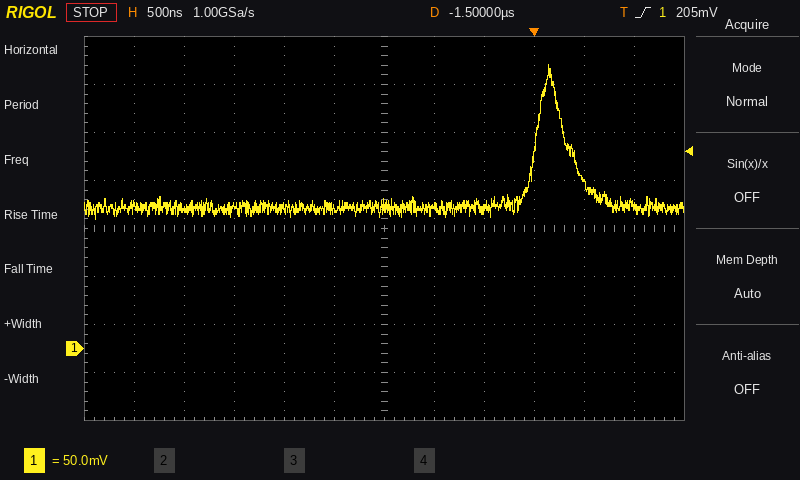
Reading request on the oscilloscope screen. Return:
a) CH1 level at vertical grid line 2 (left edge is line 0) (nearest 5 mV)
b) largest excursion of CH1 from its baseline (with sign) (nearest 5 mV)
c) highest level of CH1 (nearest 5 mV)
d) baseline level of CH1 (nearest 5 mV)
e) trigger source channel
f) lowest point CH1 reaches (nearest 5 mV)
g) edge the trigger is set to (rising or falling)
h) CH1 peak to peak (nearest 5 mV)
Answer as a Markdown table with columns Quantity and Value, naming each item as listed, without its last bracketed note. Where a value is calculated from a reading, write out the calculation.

| Quantity | Value |
|---|---|
| CH1 level at vertical grid line 2 (left edge is line 0) | 145 mV |
| largest excursion of CH1 from its baseline (with sign) | 295 mV − (145 mV) = +150 mV |
| highest level of CH1 | 295 mV |
| baseline level of CH1 | 145 mV |
| trigger source channel | CH1 |
| lowest point CH1 reaches | 135 mV |
| edge the trigger is set to | rising |
| CH1 peak to peak | 295 mV − (135 mV) = 160 mV |
